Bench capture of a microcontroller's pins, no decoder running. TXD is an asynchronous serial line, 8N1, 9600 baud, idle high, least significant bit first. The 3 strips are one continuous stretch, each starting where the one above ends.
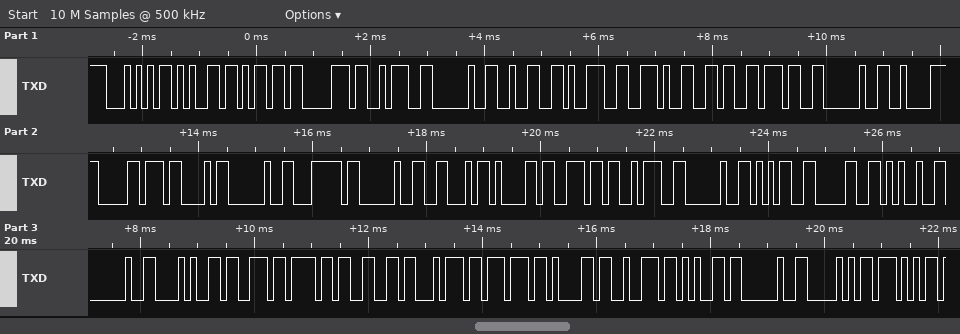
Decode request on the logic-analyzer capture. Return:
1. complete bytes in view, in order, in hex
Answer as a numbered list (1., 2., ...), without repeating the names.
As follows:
1. 54 65 6D 70 3A 20 32 39 2E 36 37 20 C2 B0 43 20 7C 20 46 61 6E 3A 20 35 30 25 20 28 73 6F 66 74 77 61 72 65 20 50 57
